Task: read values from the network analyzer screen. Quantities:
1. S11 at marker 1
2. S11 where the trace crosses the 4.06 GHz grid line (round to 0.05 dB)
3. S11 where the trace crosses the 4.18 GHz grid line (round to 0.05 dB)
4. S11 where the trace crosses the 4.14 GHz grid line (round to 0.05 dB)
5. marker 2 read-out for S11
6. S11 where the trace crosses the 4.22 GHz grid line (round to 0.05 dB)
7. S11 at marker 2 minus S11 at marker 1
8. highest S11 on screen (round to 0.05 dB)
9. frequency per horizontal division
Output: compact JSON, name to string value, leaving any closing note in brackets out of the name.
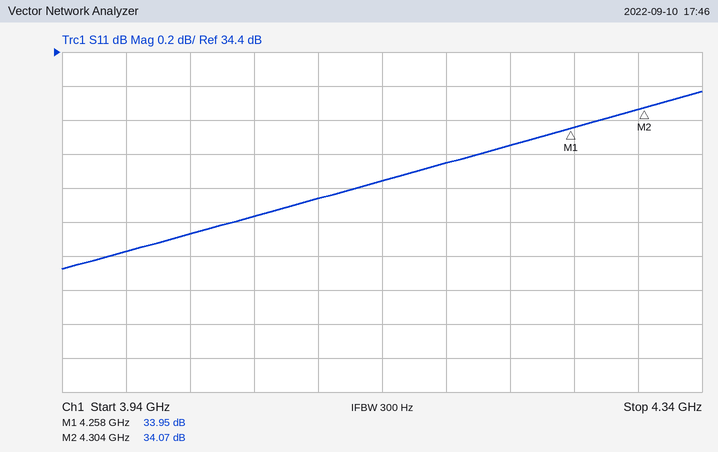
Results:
{"S11 at marker 1": "33.95 dB", "S11 where the trace crosses the 4.06 GHz grid line": "33.45 dB", "S11 where the trace crosses the 4.18 GHz grid line": "33.75 dB", "S11 where the trace crosses the 4.14 GHz grid line": "33.65 dB", "marker 2 read-out for S11": "34.07 dB", "S11 where the trace crosses the 4.22 GHz grid line": "33.85 dB", "S11 at marker 2 minus S11 at marker 1": "0.12 dB", "highest S11 on screen": "34.15 dB", "frequency per horizontal division": "40 MHz"}
